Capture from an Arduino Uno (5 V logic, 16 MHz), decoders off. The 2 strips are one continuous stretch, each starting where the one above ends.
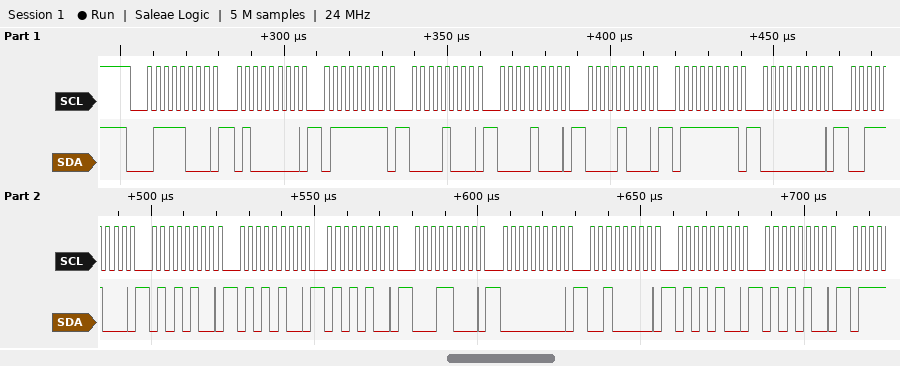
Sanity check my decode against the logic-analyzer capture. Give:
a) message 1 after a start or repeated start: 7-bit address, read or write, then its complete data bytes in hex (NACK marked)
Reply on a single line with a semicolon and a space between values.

0x3C write: 40 7F 08 08 08 7F 00 38 54 54 54 18 00 20 54 54
